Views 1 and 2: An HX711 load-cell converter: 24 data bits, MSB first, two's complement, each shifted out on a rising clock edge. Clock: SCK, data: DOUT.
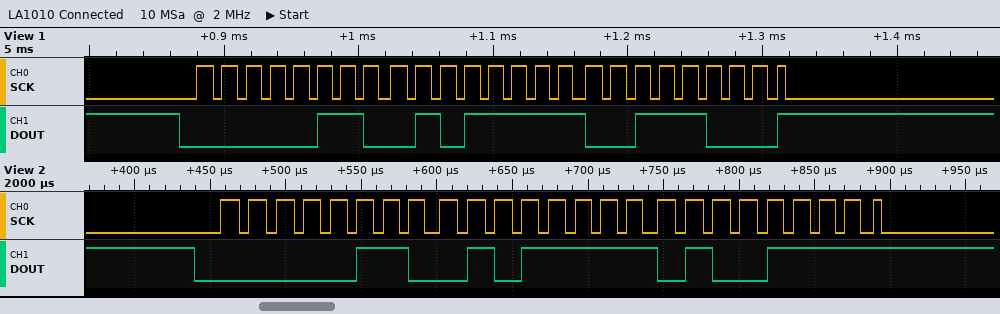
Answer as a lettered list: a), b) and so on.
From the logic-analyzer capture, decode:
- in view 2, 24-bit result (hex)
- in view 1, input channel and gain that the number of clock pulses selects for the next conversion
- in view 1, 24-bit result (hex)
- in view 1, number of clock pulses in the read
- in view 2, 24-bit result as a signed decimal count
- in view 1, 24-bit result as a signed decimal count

a) 0x065F4F
b) channel A, gain 128
c) 0x065F38
d) 25
e) 417615
f) 417592
